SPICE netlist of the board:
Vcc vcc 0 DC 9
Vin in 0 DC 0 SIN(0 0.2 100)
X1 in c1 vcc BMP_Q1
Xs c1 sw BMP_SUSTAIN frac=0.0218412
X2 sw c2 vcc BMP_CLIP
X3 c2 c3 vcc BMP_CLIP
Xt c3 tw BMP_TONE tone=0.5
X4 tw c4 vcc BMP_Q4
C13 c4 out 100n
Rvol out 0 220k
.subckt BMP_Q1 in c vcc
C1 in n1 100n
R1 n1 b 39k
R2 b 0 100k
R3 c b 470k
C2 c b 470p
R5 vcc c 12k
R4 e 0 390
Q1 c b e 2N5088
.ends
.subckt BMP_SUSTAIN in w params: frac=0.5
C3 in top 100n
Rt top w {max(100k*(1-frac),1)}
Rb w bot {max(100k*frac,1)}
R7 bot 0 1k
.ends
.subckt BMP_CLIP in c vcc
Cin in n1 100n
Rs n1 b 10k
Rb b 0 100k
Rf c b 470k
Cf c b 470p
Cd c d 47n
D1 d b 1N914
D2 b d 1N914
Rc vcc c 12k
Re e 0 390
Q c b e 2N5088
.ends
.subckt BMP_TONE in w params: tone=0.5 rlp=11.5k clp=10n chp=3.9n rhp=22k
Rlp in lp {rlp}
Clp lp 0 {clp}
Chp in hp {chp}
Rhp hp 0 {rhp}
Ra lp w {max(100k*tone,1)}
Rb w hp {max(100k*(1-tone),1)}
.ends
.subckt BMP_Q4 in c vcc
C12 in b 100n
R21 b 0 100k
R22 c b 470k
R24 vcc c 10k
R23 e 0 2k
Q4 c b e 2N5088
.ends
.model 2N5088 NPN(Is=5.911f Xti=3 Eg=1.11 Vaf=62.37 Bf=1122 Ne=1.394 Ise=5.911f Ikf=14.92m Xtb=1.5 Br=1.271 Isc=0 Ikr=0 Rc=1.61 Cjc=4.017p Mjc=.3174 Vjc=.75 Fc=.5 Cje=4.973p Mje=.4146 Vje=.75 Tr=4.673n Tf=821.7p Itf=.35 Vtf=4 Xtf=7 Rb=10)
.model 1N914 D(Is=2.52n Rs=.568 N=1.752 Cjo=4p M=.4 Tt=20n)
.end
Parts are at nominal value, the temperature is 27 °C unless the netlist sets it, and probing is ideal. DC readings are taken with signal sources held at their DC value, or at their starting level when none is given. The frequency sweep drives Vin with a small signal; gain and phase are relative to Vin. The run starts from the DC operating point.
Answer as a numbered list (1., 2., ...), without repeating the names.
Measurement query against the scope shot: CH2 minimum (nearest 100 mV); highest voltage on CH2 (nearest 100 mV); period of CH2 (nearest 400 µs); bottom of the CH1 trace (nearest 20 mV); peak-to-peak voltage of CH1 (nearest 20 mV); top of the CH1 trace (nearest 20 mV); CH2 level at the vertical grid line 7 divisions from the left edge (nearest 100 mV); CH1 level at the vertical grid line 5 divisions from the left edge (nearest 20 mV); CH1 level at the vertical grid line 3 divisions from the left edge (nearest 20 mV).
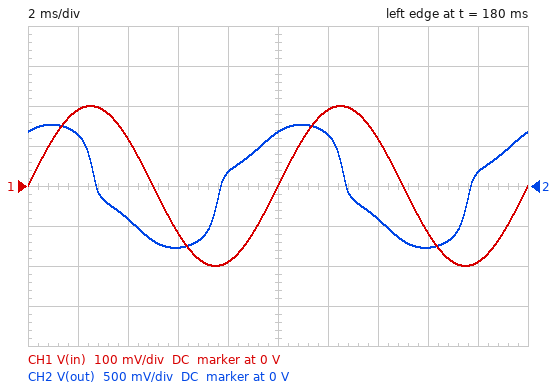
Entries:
1. -800 mV
2. 800 mV
3. 10.0 ms
4. -200 mV
5. 400 mV
6. 200 mV
7. -400 mV
8. 0 V
9. -120 mV
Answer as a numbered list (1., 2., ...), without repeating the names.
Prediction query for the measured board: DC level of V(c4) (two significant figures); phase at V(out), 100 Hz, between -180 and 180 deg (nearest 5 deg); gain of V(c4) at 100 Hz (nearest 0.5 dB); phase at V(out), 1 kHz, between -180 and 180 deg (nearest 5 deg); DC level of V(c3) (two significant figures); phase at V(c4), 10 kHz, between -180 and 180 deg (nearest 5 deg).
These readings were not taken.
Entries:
1. 6.5 V
2. 80 deg
3. 28.5 dB
4. -95 deg
5. 4.6 V
6. 135 deg
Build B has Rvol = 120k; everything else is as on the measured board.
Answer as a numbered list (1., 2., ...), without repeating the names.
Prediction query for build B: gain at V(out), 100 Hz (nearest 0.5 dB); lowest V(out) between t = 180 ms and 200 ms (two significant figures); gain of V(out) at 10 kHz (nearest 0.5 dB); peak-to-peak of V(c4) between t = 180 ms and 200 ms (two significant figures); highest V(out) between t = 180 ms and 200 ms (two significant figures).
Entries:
1. 28.0 dB
2. -740 mV
3. -15.0 dB
4. 1.5 V
5. 730 mV
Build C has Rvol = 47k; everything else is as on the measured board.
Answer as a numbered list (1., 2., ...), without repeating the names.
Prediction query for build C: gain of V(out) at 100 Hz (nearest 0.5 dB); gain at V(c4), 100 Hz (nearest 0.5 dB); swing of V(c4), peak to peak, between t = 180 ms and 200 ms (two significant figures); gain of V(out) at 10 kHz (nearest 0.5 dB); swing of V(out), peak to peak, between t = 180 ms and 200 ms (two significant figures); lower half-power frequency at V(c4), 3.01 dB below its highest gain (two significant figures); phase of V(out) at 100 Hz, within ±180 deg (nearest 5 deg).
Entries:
1. 27.0 dB
2. 27.5 dB
3. 1.4 V
4. -15.5 dB
5. 1.3 V
6. 72 Hz
7. 90 deg
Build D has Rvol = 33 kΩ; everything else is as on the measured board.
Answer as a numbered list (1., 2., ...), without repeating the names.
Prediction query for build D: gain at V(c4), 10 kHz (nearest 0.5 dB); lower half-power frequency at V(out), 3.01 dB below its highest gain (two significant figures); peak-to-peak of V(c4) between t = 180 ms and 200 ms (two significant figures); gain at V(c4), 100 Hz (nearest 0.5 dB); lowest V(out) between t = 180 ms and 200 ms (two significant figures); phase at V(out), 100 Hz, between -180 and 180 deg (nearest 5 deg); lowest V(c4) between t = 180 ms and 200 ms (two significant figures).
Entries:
1. -16.0 dB
2. 83 Hz
3. 1.4 V
4. 27.0 dB
5. -580 mV
6. 95 deg
7. 5.8 V
